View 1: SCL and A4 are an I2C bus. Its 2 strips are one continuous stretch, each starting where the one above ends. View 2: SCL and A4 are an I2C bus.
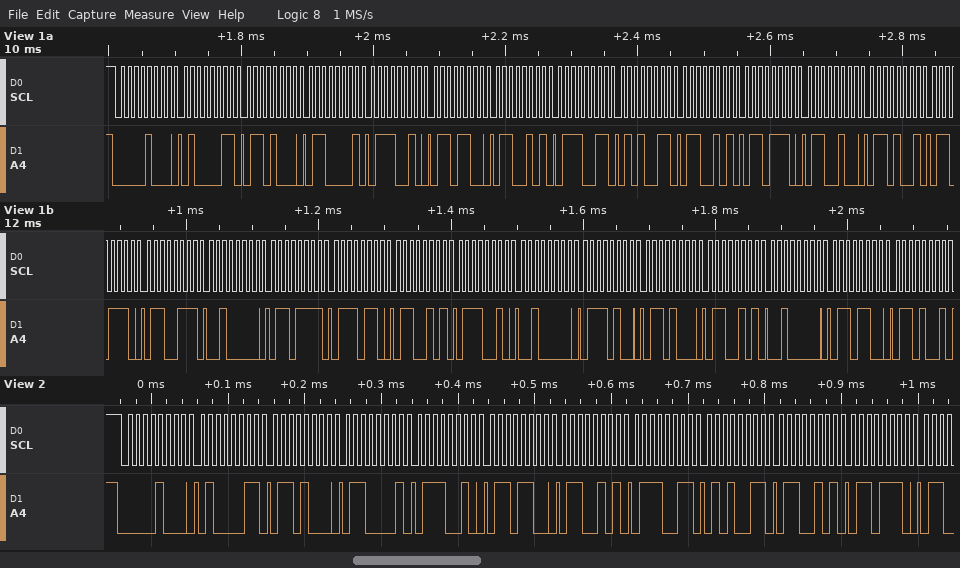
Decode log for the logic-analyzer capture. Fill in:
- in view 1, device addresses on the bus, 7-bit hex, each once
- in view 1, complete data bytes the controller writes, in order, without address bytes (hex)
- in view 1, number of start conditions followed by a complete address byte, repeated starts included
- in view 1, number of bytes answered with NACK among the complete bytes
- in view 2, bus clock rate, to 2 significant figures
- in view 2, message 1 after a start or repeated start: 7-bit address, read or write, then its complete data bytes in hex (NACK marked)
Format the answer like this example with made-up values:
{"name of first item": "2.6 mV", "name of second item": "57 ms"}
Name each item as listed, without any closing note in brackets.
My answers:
{"in view 1, device addresses on the bus, 7-bit hex, each once": "0x04", "in view 1, complete data bytes the controller writes, in order, without address bytes": "43 68 61 72 6C 65 73 53 65 6E 64 69 6E 67 20 6F 76 65 72 20 74 68 65 20 6C 69", "in view 1, number of start conditions followed by a complete address byte, repeated starts included": "1", "in view 1, number of bytes answered with NACK among the complete bytes": "0", "in view 2, bus clock rate, to 2 significant figures": "100 kHz", "in view 2, message 1 after a start or repeated start: 7-bit address, read or write, then its complete data bytes in hex": "0x04 write: 43 68 61 72 6C 65 73 53 65 6E"}
